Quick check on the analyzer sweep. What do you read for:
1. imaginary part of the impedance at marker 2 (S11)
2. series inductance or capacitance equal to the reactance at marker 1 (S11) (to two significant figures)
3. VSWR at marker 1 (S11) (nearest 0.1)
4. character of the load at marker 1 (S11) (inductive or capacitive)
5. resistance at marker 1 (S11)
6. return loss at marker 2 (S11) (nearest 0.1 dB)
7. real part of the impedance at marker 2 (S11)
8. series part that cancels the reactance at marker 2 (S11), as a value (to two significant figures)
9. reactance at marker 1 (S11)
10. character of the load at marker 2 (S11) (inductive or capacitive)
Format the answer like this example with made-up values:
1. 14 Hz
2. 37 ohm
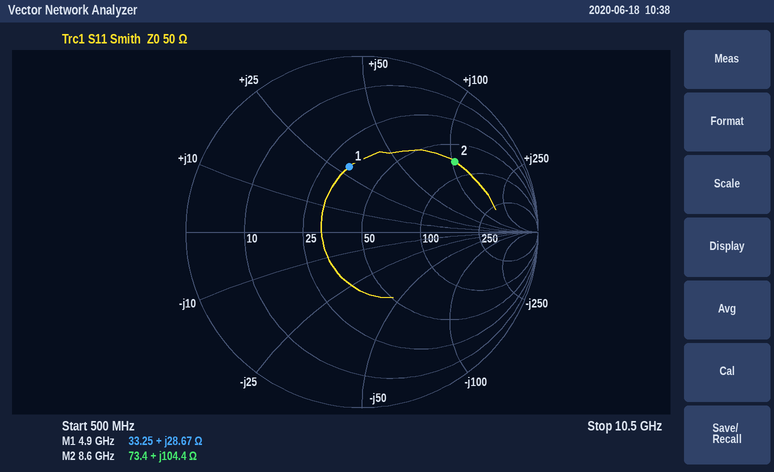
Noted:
1. +104.4 Ω
2. 930 pH
3. 2.2
4. inductive
5. 33.25 Ω
6. 3.6 dB
7. 73.4 Ω
8. 180 fF
9. +28.67 Ω
10. inductive
